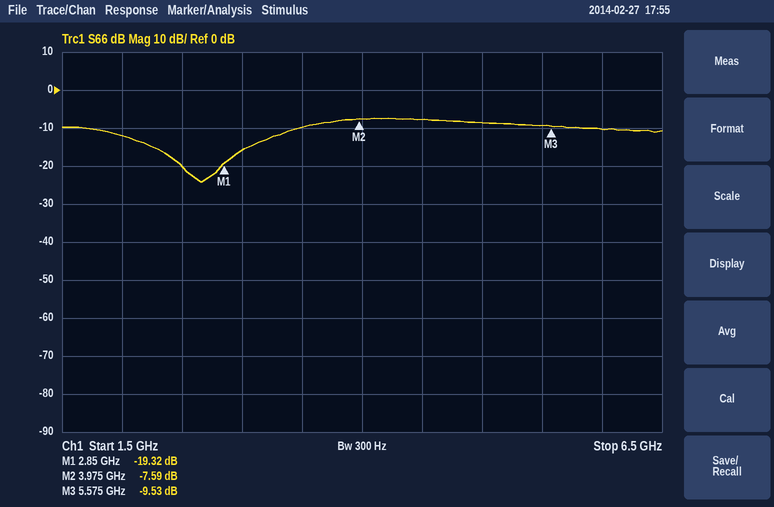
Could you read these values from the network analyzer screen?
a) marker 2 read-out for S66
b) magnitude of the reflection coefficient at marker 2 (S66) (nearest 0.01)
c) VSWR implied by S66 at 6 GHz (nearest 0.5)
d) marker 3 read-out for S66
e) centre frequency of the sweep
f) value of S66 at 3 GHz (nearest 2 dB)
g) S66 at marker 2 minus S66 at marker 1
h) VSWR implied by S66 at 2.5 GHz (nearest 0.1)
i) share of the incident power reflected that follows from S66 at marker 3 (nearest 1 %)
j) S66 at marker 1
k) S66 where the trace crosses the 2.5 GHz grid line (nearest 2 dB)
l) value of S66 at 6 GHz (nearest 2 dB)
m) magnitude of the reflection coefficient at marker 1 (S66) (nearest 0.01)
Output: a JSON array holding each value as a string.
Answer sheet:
["-7.59 dB", "0.42", "2.0", "-9.53 dB", "4 GHz", "-16 dB", "11.73 dB", "1.2", "11 %", "-19.32 dB", "-20 dB", "-10 dB", "0.11"]
